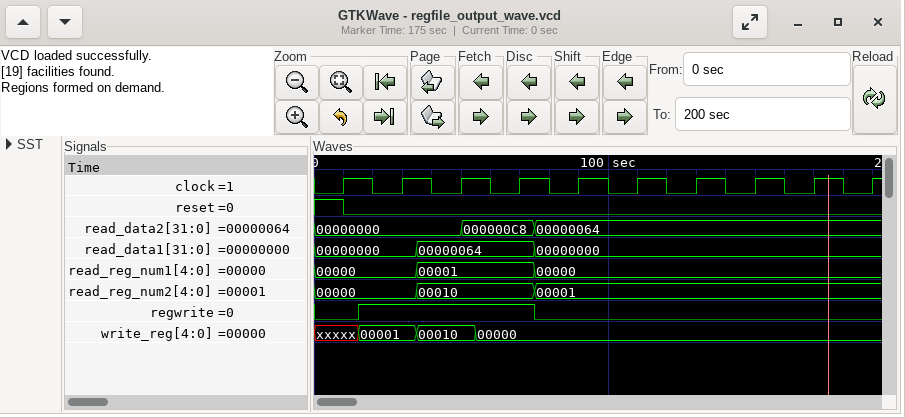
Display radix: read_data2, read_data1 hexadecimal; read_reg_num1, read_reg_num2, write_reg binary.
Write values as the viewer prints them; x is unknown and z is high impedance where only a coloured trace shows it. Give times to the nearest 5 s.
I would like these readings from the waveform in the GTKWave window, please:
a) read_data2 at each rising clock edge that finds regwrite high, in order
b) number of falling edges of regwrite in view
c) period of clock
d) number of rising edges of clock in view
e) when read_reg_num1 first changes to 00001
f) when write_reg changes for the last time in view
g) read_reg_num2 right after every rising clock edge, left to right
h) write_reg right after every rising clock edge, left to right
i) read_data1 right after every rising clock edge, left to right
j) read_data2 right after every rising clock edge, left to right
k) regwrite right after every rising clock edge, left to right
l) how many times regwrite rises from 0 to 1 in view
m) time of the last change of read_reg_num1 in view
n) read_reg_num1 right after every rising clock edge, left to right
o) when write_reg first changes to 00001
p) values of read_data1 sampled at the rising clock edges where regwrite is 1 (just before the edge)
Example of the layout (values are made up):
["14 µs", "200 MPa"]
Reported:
["00000000, 00000000, 000000C8", "1", "20 s", "10", "35 s", "55 s", "00000, 00000, 00010, 00010, 00001, 00001, 00001, 00001, 00001, 00001", "xxxxx, 00001, 00010, 00000, 00000, 00000, 00000, 00000, 00000, 00000", "00000000, 00000000, 00000064, 00000064, 00000000, 00000000, 00000000, 00000000, 00000000, 00000000", "00000000, 00000000, 000000C8, 000000C8, 00000064, 00000064, 00000064, 00000064, 00000064, 00000064", "0 1 1 1 0 0 0 0 0 0", "1", "75 s", "00000, 00000, 00001, 00001, 00000, 00000, 00000, 00000, 00000, 00000", "15 s", "00000000, 00000064, 00000064"]
